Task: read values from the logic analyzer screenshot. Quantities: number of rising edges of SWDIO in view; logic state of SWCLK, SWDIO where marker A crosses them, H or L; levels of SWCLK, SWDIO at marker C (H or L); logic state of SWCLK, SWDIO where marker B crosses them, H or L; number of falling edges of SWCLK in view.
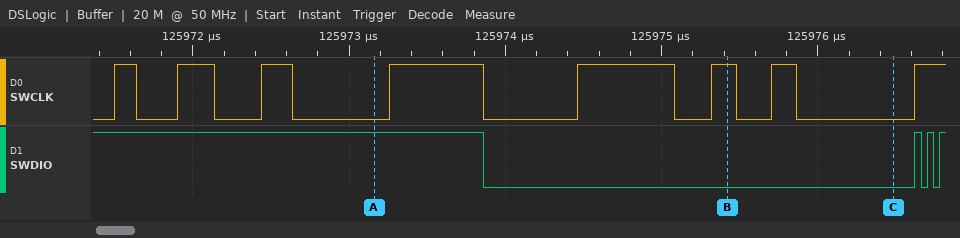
3
SWCLK=L, SWDIO=H
SWCLK=L, SWDIO=L
SWCLK=H, SWDIO=L
7
